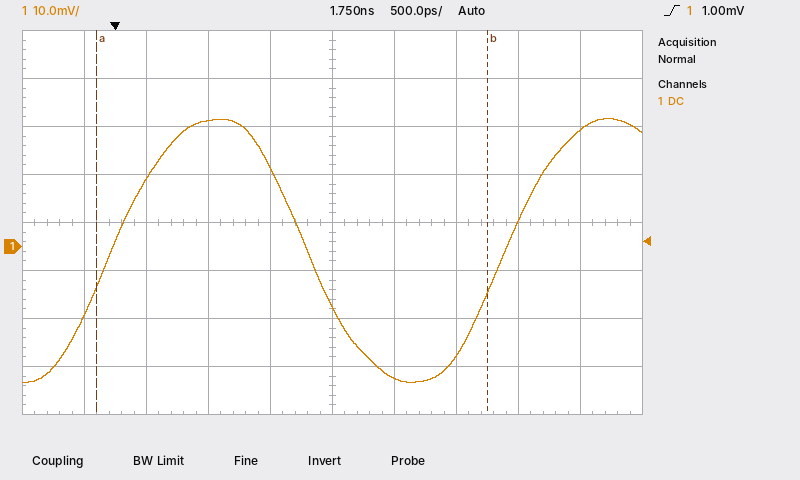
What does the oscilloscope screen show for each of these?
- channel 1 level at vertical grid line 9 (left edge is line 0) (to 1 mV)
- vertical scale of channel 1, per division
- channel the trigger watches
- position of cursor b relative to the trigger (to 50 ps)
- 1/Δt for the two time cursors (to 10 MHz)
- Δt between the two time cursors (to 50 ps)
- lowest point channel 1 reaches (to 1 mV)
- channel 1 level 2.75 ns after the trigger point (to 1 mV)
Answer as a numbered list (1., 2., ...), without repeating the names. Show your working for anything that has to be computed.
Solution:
1. 24 mV
2. 10 mV
3. channel 1
4. +3.00 ns
5. 1 / 3.15 ns ≈ 320 MHz
6. 3.15 ns
7. -28 mV
8. -23 mV
